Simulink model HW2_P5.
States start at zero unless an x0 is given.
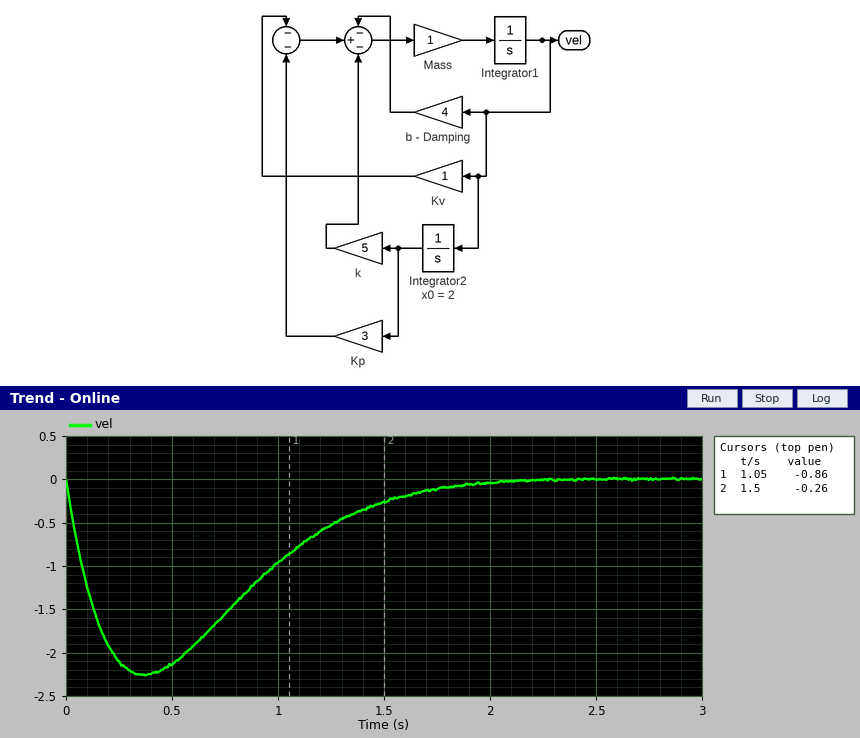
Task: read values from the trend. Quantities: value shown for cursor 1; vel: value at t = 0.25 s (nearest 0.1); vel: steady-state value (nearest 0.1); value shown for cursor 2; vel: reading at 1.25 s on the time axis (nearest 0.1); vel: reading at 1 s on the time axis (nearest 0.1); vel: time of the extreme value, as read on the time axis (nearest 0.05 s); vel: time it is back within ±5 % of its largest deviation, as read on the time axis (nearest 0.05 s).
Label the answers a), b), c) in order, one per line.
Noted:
a) -0.86
b) -2.1
c) 0.0
d) -0.26
e) -0.5
f) -1.0
g) 0.35 s
h) 1.75 s
